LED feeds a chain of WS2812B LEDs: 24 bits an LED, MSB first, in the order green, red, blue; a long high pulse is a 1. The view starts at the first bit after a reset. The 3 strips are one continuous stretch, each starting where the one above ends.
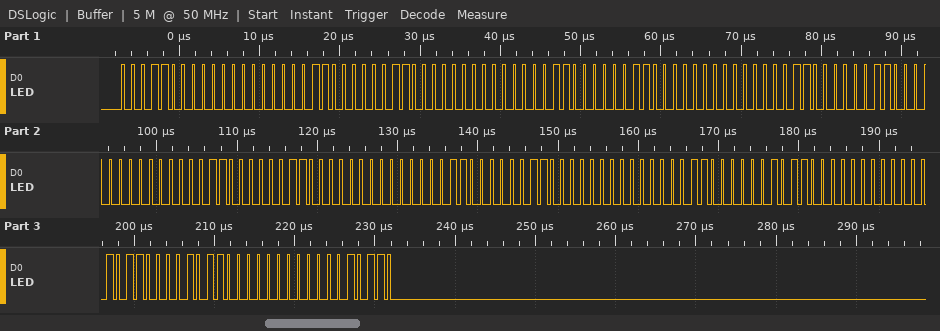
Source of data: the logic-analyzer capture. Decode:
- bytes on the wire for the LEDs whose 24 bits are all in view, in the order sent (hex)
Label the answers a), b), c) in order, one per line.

a) 18 00 18 18 00 18 18 00 18 18 00 18 18 00 18 18 00 18 16 00 16 16 00 16
